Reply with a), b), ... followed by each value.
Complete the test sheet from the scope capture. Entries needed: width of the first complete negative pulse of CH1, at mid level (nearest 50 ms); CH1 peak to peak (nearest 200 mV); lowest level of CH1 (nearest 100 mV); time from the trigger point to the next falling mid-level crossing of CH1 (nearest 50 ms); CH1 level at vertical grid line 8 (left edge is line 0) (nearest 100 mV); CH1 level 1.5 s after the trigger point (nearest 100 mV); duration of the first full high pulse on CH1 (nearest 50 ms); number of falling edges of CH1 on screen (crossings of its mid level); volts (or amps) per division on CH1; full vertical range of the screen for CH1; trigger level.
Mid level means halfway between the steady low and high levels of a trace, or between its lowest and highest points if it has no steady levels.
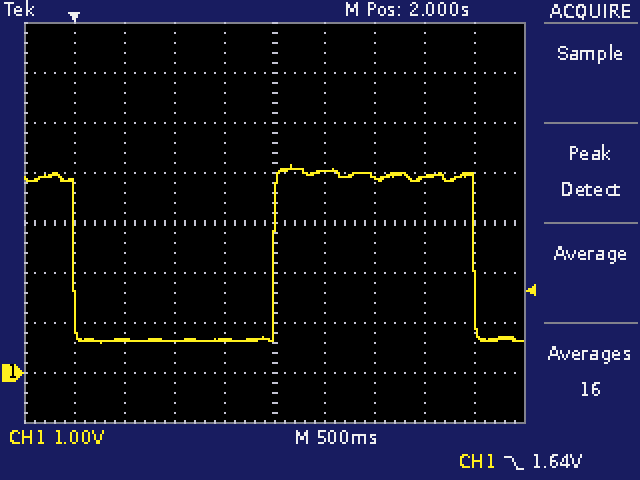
a) 2.00 s
b) 3.6 V
c) 600 mV
d) 4.00 s
e) 3.9 V
f) 700 mV
g) 2.00 s
h) 2
i) 1 V
j) 8 V
k) 1.64 V
